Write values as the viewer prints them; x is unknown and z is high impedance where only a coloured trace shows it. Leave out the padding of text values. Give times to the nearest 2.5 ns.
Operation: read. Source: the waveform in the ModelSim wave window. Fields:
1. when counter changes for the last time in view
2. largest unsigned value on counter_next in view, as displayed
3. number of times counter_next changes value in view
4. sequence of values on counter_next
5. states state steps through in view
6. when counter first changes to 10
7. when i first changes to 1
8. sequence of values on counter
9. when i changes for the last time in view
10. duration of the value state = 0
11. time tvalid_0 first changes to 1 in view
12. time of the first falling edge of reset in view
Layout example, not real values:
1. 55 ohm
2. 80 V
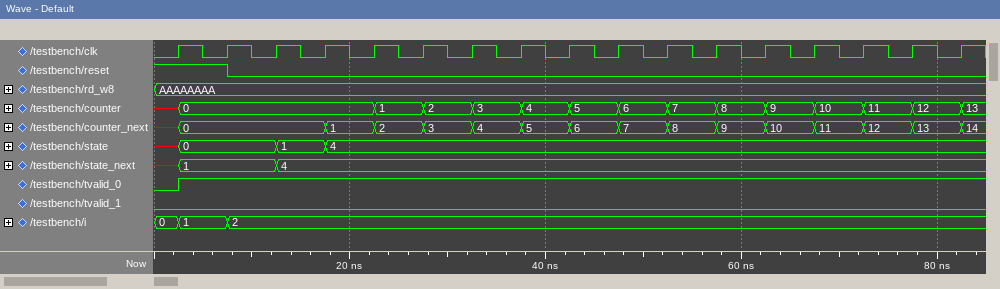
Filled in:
1. 82.5 ns
2. 14
3. 15
4. x, 0, 1, 2, 3, 4, 5, 6, 7, 8, 9, 10, 11, 12, 13, 14
5. x, 0, 1, 4
6. 67.5 ns
7. 2.5 ns
8. x, 0, 1, 2, 3, 4, 5, 6, 7, 8, 9, 10, 11, 12, 13
9. 7.5 ns
10. 10 ns
11. 2.5 ns
12. 7.5 ns
